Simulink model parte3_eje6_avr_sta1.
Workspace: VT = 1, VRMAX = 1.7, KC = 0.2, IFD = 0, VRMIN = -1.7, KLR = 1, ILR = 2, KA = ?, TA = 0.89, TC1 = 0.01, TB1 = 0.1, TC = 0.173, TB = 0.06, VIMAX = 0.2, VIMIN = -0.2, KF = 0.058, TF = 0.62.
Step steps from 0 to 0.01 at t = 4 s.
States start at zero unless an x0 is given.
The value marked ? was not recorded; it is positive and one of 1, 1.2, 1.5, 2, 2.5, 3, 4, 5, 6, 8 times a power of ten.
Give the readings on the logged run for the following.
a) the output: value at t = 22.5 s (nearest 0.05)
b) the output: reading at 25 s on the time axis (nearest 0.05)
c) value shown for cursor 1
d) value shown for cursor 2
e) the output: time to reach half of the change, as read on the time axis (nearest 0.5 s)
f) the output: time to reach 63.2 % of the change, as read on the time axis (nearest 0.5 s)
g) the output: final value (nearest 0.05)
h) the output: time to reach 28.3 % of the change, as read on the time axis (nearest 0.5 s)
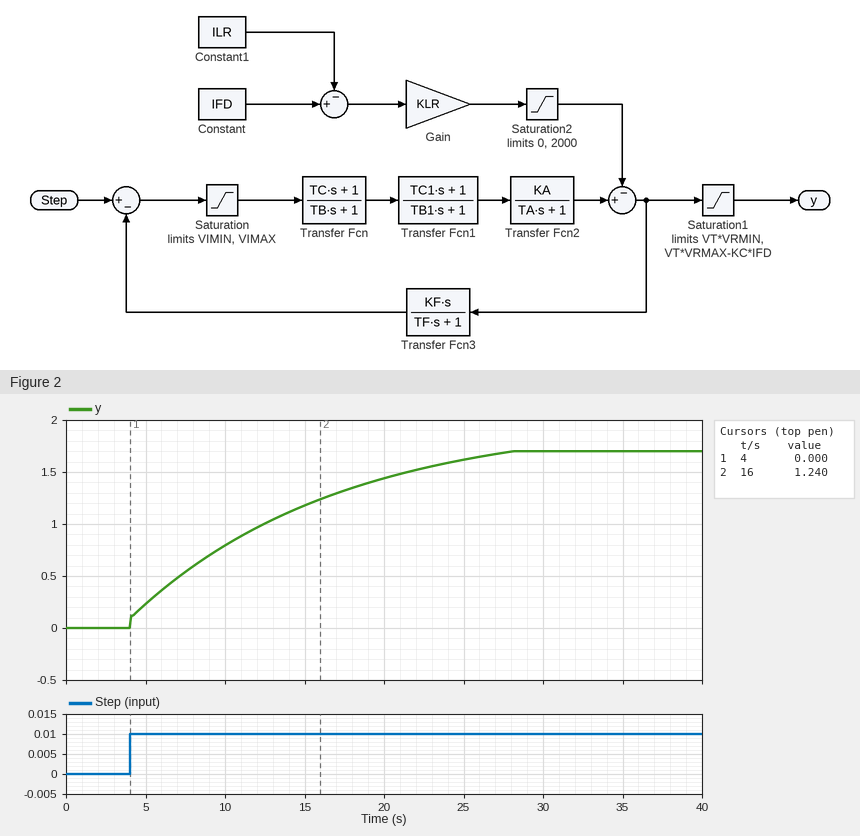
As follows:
1.55
1.60
0.000
1.240
10.5 s
13.5 s
1.70
7.0 s
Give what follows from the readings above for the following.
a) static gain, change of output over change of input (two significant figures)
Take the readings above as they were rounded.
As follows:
170
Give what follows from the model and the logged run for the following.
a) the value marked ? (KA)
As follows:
200
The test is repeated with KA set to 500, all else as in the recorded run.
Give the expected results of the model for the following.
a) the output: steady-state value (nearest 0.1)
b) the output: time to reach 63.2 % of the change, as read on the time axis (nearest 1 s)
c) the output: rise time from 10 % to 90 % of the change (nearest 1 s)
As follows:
1.7
11 s
10 s
